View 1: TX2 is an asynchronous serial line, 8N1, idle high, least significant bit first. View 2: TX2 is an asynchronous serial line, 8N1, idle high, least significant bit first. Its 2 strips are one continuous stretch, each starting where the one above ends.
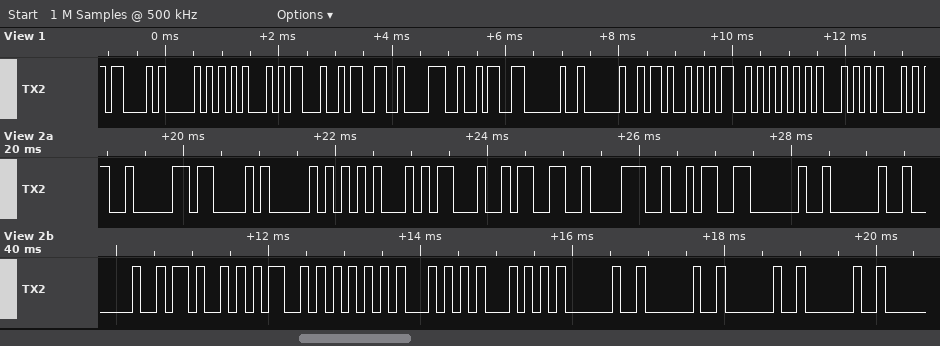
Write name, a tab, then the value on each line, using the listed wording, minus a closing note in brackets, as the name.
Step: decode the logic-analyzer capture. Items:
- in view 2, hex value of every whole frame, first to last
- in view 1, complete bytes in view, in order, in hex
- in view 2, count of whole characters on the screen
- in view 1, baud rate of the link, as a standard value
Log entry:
in view 2, hex value of every whole frame, first to last	82 43 50 45 23 33 38 9A 20 20 20 4B 4D 55 54 54 20 20 20 20
in view 1, complete bytes in view, in order, in hex	43 50 45 23 33 38 9A 20 20 4B 4D 55 54
in view 2, count of whole characters on the screen	20
in view 1, baud rate of the link, as a standard value	9600 baud
